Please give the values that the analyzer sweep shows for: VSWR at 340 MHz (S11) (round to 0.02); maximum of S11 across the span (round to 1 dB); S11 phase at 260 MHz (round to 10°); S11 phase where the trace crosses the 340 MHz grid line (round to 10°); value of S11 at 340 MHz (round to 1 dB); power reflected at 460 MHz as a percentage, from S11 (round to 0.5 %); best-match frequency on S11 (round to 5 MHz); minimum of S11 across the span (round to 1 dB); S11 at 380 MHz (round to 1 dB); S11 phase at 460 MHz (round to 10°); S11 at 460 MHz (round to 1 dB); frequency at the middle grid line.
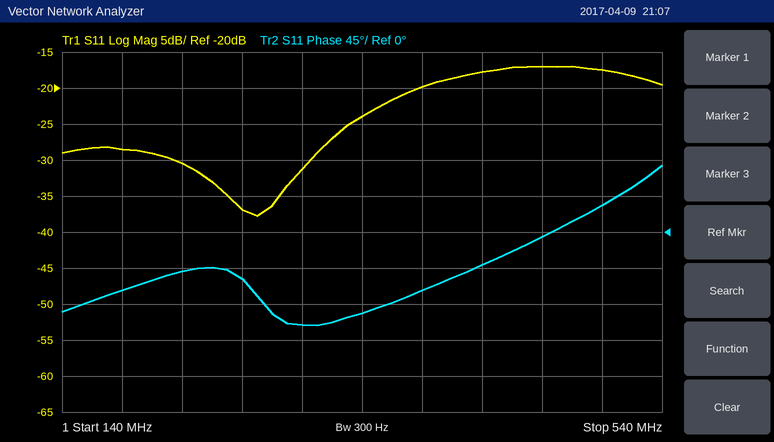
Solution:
1.14
-17 dB
-60°
-100°
-24 dB
2.0 %
270 MHz
-38 dB
-20 dB
-10°
-17 dB
340 MHz
